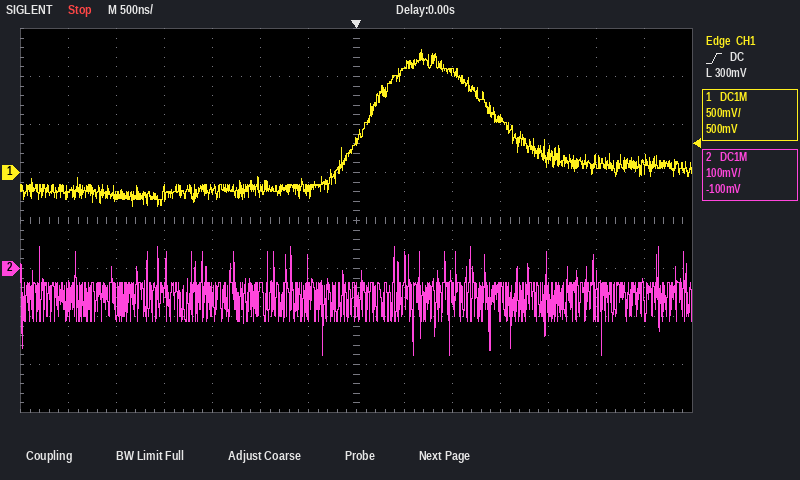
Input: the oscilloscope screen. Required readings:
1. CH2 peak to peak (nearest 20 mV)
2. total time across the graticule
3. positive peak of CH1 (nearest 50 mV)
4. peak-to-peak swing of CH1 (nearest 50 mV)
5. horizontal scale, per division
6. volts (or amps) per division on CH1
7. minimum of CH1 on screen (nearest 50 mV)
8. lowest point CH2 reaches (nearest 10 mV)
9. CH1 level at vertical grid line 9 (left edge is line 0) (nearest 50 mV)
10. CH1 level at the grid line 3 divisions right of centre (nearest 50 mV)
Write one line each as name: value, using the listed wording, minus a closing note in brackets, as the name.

CH2 peak to peak: 220 mV
total time across the graticule: 7 µs
positive peak of CH1: 1.30 V
peak-to-peak swing of CH1: 1.65 V
horizontal scale, per division: 500 ns
volts (or amps) per division on CH1: 500 mV
minimum of CH1 on screen: -350 mV
lowest point CH2 reaches: -180 mV
CH1 level at vertical grid line 9 (left edge is line 0): 1.05 V
CH1 level at the grid line 3 divisions right of centre: 550 mV
